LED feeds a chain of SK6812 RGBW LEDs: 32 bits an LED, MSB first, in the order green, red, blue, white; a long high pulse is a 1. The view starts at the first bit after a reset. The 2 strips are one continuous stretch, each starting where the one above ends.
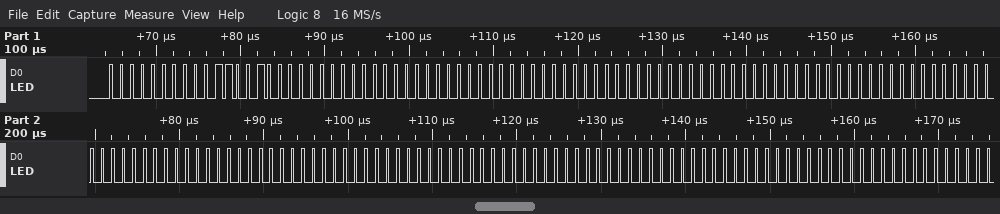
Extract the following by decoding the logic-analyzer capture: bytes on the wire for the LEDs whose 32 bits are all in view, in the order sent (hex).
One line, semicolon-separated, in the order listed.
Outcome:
00 32 00 00 00 00 00 00 00 00 00 00 00 00 00 00 00 00 00 00
